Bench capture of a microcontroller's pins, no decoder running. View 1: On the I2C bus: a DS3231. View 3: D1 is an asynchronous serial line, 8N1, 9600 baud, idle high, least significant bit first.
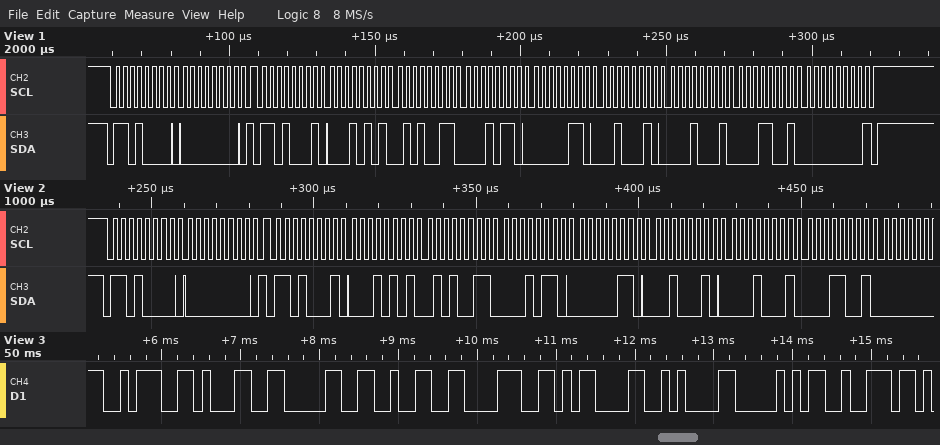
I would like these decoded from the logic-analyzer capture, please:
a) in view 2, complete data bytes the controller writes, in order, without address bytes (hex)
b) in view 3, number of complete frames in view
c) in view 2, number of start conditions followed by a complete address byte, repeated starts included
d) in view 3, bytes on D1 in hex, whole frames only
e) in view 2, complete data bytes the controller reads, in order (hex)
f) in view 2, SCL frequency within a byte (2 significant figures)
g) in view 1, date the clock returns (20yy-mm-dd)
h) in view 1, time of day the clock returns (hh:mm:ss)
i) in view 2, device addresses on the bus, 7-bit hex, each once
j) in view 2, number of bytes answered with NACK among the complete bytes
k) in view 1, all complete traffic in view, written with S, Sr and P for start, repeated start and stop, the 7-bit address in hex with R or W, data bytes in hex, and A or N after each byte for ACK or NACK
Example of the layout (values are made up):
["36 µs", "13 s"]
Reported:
["00", "9", "2", "3A 31 30 32 38 0D 0A 50 72", "15 53 16 06 22 11 19", "400 kHz", "2019-11-22", "16:53:15", "0x68", "0", "S 68W A 00 A Sr 68R A 15 A 53 A 16 A 06 A 22 A 11 A 19 A 00 N P"]
